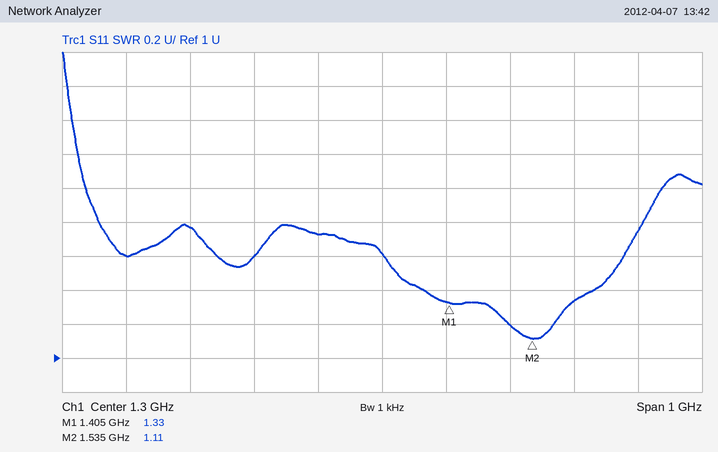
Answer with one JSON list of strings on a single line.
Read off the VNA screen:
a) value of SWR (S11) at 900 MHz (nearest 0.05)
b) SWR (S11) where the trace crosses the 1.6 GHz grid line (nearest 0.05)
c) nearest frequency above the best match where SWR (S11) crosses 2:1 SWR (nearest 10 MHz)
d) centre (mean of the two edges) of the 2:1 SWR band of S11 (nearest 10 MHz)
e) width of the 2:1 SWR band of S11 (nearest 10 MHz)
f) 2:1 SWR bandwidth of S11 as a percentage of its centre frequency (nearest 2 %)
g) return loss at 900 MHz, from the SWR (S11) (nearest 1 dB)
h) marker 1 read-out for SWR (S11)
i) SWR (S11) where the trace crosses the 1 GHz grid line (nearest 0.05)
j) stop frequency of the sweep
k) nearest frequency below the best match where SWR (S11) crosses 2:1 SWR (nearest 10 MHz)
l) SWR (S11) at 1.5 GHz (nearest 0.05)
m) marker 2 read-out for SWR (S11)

["1.60", "1.35", "1.74 GHz", "1.29 GHz", "900 MHz", "70 %", "13 dB", "1.33", "1.75", "1.8 GHz", "840 MHz", "1.20", "1.11"]
